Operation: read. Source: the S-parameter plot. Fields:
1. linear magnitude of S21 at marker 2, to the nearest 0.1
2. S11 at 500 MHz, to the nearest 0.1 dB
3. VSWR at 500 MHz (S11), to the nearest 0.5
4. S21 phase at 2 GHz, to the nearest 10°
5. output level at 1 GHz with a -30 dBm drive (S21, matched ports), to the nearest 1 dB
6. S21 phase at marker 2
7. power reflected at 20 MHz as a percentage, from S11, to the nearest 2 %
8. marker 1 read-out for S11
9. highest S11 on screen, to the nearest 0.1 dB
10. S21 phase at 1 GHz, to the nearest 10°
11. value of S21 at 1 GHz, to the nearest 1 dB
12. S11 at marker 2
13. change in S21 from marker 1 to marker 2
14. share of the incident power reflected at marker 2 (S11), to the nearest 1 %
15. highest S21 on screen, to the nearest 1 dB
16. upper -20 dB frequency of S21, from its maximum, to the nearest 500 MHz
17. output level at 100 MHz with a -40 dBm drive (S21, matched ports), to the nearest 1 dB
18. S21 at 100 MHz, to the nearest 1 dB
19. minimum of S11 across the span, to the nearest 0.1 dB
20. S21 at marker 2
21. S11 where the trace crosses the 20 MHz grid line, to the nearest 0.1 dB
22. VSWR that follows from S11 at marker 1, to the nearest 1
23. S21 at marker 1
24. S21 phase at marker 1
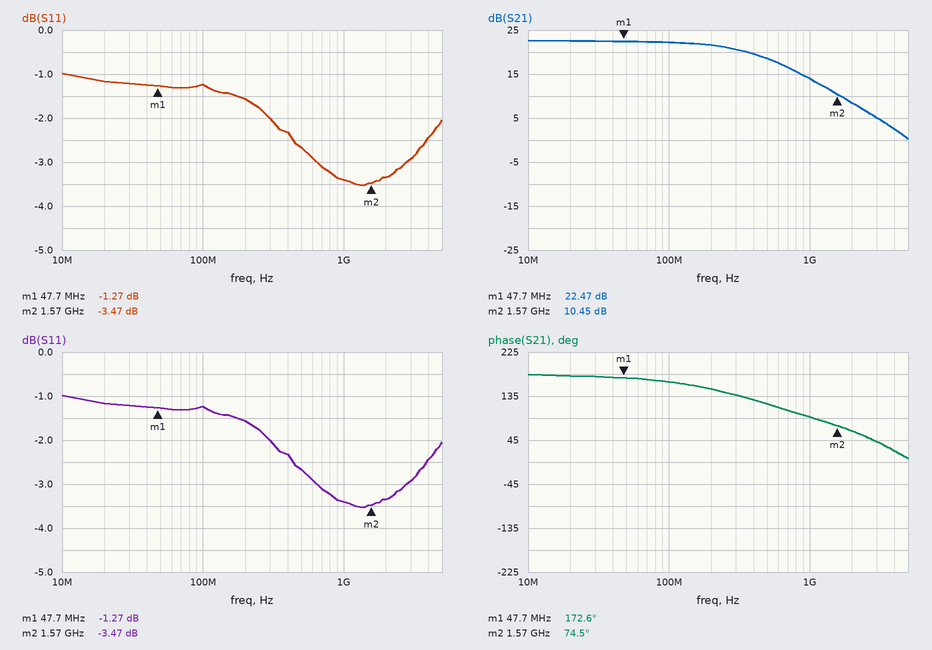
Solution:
3.3
-2.7 dB
6.5
60°
-16 dBm
74.5°
76 %
-1.27 dB
-1.0 dB
90°
14 dB
-3.47 dB
-12.02 dB
45 %
23 dB
4.0 GHz
-18 dBm
22 dB
-3.5 dB
10.45 dB
-1.2 dB
14
22.47 dB
172.6°
